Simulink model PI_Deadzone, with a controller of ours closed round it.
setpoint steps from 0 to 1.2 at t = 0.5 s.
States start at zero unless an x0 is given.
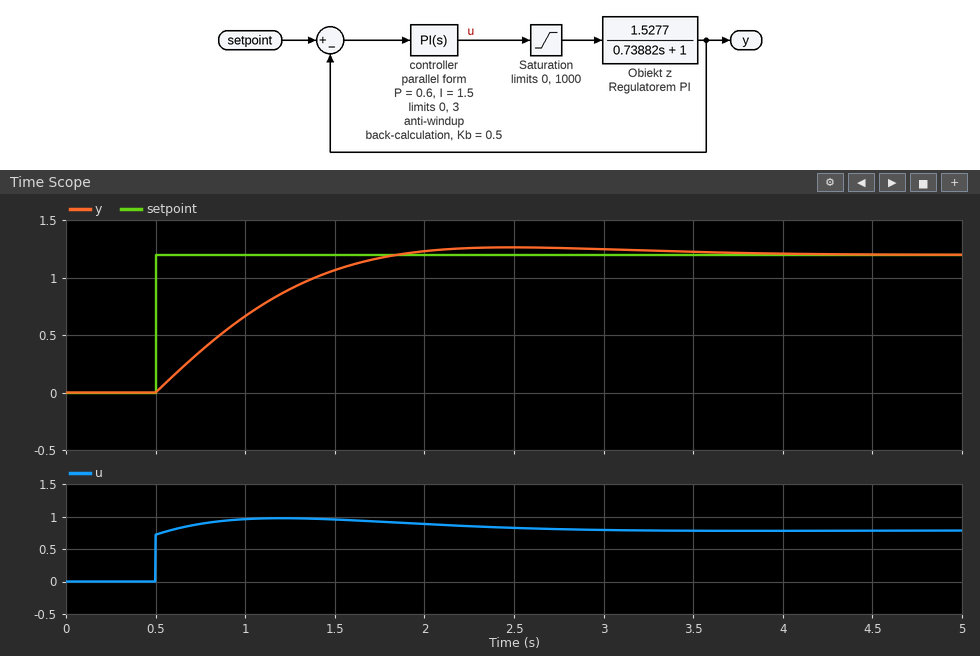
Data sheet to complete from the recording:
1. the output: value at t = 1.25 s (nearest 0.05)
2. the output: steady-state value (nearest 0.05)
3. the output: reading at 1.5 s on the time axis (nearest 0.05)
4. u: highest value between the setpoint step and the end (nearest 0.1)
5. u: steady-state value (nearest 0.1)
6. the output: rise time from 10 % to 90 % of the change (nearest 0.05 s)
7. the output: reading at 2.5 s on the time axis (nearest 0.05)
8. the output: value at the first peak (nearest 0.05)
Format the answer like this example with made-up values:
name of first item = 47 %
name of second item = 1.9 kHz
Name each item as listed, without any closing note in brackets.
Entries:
the output: value at t = 1.25 s = 0.90
the output: steady-state value = 1.20
the output: reading at 1.5 s on the time axis = 1.05
u: highest value between the setpoint step and the end = 1.0
u: steady-state value = 0.8
the output: rise time from 10 % to 90 % of the change = 0.95 s
the output: reading at 2.5 s on the time axis = 1.25
the output: value at the first peak = 1.25
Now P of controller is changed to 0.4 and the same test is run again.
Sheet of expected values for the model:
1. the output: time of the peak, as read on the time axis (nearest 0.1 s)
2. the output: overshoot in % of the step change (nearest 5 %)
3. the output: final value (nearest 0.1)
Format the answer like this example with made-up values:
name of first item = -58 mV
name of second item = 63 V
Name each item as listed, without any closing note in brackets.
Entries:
the output: time of the peak, as read on the time axis = 2.4 s
the output: overshoot in % of the step change = 10 %
the output: final value = 1.2
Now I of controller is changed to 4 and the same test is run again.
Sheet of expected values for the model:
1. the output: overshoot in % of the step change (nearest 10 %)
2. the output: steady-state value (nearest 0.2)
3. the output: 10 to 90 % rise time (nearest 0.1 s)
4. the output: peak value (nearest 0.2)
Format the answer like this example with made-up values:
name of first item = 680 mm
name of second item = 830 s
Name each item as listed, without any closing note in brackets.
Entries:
the output: overshoot in % of the step change = 20 %
the output: steady-state value = 1.2
the output: 10 to 90 % rise time = 0.5 s
the output: peak value = 1.4
